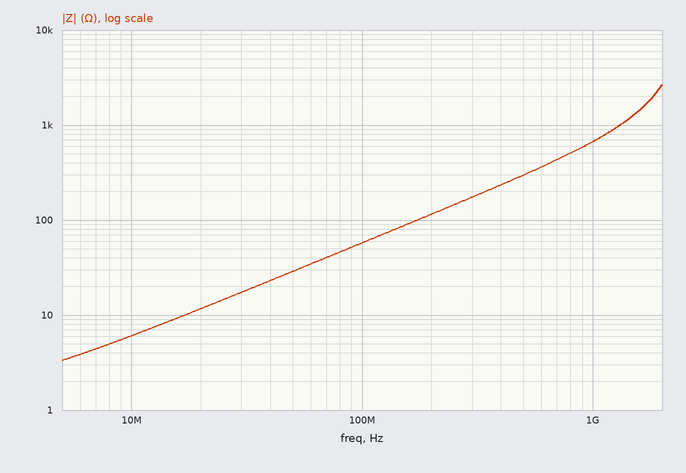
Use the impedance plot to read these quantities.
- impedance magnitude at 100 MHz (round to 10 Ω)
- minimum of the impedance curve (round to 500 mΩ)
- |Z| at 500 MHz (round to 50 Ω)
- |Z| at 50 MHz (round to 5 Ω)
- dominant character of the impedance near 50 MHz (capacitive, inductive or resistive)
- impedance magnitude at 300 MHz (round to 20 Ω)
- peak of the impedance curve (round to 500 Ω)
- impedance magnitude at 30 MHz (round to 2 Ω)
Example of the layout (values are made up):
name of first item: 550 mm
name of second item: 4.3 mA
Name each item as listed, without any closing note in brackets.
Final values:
impedance magnitude at 100 MHz: 60 Ω
minimum of the impedance curve: 3.5 Ω
|Z| at 500 MHz: 300 Ω
|Z| at 50 MHz: 30 Ω
dominant character of the impedance near 50 MHz: inductive
impedance magnitude at 300 MHz: 180 Ω
peak of the impedance curve: 2.5 kΩ
impedance magnitude at 30 MHz: 18 Ω
